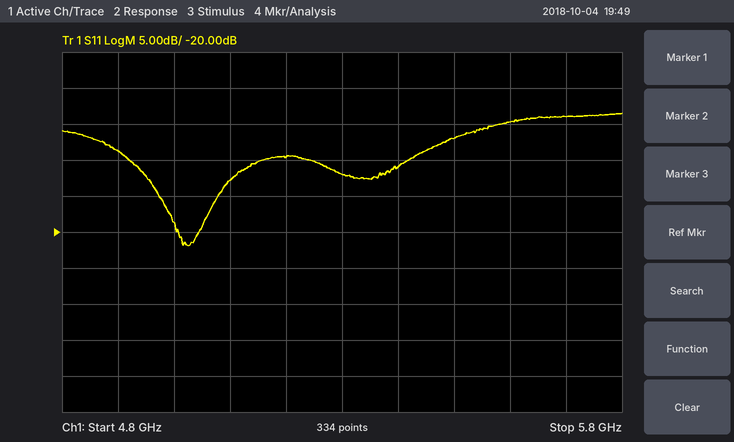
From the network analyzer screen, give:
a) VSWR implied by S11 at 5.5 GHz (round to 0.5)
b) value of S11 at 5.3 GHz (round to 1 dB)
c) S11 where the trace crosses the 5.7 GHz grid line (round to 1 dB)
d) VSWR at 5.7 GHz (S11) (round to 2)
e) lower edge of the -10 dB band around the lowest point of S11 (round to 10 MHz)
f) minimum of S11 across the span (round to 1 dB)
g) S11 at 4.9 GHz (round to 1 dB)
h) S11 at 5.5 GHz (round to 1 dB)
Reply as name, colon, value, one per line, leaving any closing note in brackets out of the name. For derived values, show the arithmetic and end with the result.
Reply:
VSWR implied by S11 at 5.5 GHz: |Γ| = 10^(-7/20) = 0.4467; VSWR = (1 + 0.4467)/(1 − 0.4467) ≈ 2.61, so 2.5 to the nearest 0.5
value of S11 at 5.3 GHz: -12 dB
S11 where the trace crosses the 5.7 GHz grid line: -4 dB
VSWR at 5.7 GHz (S11): |Γ| = 10^(-4/20) = 0.6310; VSWR = (1 + 0.6310)/(1 − 0.6310) ≈ 4
lower edge of the -10 dB band around the lowest point of S11: 4.92 GHz
minimum of S11 across the span: -22 dB
S11 at 4.9 GHz: -9 dB
S11 at 5.5 GHz: -7 dB
